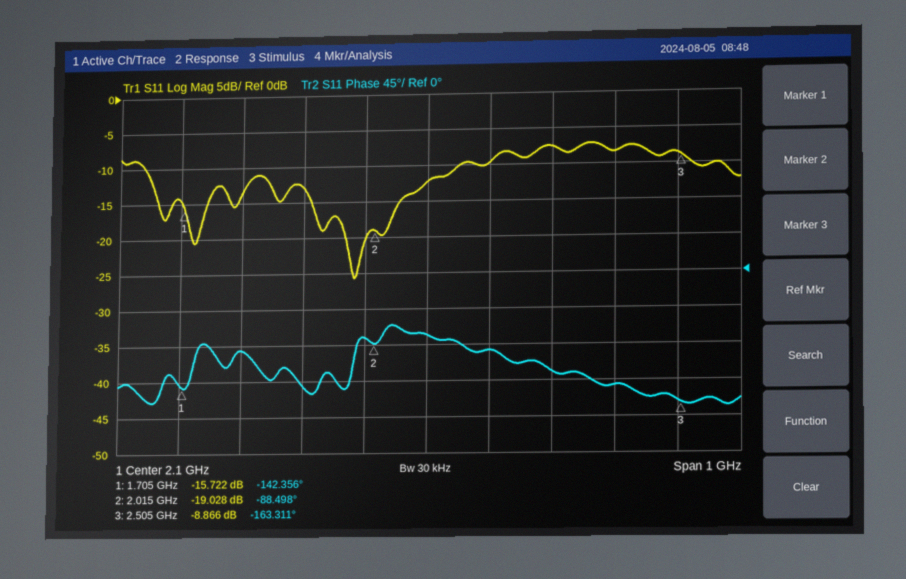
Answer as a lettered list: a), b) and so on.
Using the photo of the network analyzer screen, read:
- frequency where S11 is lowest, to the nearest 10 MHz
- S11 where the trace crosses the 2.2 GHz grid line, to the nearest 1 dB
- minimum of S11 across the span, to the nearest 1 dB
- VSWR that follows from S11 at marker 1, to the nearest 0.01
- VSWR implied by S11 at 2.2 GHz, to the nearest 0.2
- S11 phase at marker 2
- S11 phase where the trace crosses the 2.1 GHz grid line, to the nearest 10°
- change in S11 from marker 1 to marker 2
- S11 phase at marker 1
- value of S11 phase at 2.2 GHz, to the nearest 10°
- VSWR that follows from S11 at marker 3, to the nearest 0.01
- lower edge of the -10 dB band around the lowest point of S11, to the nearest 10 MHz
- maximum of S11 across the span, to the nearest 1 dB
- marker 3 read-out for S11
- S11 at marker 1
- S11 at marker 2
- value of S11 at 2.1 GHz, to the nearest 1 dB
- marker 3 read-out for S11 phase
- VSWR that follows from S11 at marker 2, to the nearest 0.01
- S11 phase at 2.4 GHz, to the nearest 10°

a) 1.98 GHz
b) -10 dB
c) -26 dB
d) 1.39
e) 2.0
f) -88.498°
g) -80°
h) -3.306 dB
i) -142.356°
j) -100°
k) 2.13
l) 1.64 GHz
m) -7 dB
n) -8.866 dB
o) -15.722 dB
p) -19.028 dB
q) -12 dB
r) -163.311°
s) 1.25
t) -140°
